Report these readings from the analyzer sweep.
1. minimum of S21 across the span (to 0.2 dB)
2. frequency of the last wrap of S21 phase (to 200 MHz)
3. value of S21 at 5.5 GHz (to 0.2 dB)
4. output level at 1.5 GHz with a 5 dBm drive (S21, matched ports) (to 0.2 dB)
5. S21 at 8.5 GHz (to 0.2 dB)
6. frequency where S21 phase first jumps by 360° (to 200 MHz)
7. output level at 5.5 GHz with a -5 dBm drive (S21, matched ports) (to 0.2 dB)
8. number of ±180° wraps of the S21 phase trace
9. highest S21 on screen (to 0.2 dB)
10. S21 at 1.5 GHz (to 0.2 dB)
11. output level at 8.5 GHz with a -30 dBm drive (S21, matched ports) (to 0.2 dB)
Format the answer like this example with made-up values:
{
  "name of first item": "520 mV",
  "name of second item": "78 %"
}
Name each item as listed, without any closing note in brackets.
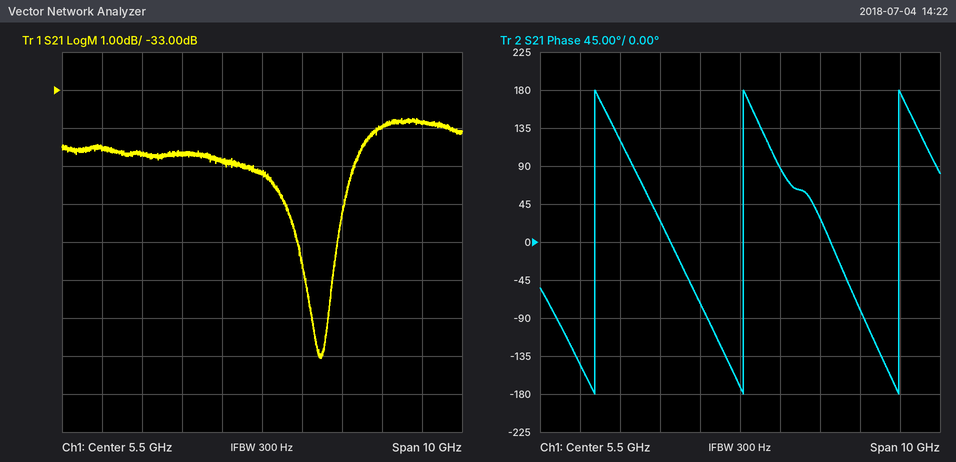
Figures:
{
  "minimum of S21 across the span": "-40.0 dB",
  "frequency of the last wrap of S21 phase": "9.4 GHz",
  "value of S21 at 5.5 GHz": "-35.2 dB",
  "output level at 1.5 GHz with a 5 dBm drive (S21, matched ports)": "-29.6 dBm",
  "S21 at 8.5 GHz": "-34.0 dB",
  "frequency where S21 phase first jumps by 360°": "1.8 GHz",
  "output level at 5.5 GHz with a -5 dBm drive (S21, matched ports)": "-40.2 dBm",
  "number of ±180° wraps of the S21 phase trace": "3",
  "highest S21 on screen": "-33.8 dB",
  "S21 at 1.5 GHz": "-34.6 dB",
  "output level at 8.5 GHz with a -30 dBm drive (S21, matched ports)": "-64.0 dBm"
}
